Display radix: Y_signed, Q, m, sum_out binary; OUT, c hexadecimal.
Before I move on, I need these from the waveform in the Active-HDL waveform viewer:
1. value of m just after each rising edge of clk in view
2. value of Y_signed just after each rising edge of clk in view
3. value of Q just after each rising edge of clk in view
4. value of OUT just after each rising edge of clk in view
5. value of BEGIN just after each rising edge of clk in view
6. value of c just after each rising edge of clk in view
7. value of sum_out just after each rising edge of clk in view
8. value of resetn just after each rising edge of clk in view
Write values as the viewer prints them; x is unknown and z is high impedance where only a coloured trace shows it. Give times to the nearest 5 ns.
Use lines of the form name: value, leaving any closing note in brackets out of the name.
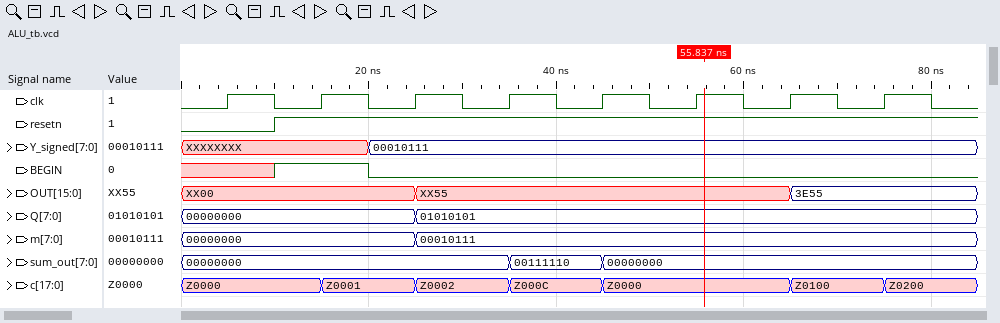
value of m just after each rising edge of clk in view: 00000000, 00000000, 00010111, 00010111, 00010111, 00010111, 00010111, 00010111
value of Y_signed just after each rising edge of clk in view: XXXXXXXX, XXXXXXXX, 00010111, 00010111, 00010111, 00010111, 00010111, 00010111
value of Q just after each rising edge of clk in view: 00000000, 00000000, 01010101, 01010101, 01010101, 01010101, 01010101, 01010101
value of OUT just after each rising edge of clk in view: XX00, XX00, XX55, XX55, XX55, XX55, 3E55, 3E55
value of BEGIN just after each rising edge of clk in view: x 1 0 0 0 0 0 0
value of c just after each rising edge of clk in view: Z0000, Z0001, Z0002, Z000C, Z0000, Z0000, Z0100, Z0200
value of sum_out just after each rising edge of clk in view: 00000000, 00000000, 00000000, 00111110, 00000000, 00000000, 00000000, 00000000
value of resetn just after each rising edge of clk in view: 0 1 1 1 1 1 1 1
